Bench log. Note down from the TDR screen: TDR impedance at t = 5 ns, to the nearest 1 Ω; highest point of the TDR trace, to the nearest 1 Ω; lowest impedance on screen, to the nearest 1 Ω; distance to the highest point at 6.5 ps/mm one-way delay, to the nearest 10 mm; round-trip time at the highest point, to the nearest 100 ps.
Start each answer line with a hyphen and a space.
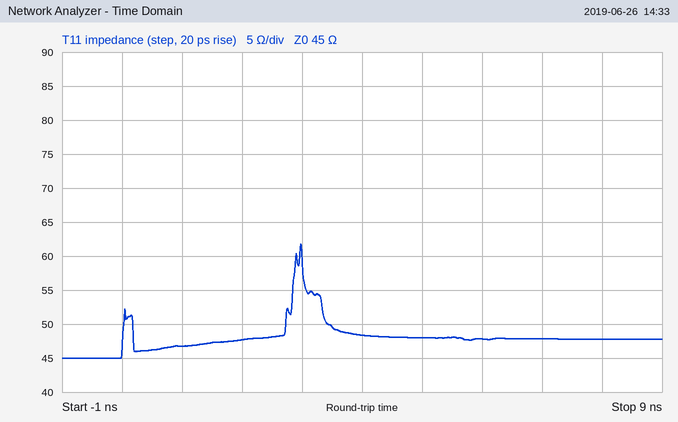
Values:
- 48 Ω
- 62 Ω
- 45 Ω
- 230 mm
- 3.0 ns
